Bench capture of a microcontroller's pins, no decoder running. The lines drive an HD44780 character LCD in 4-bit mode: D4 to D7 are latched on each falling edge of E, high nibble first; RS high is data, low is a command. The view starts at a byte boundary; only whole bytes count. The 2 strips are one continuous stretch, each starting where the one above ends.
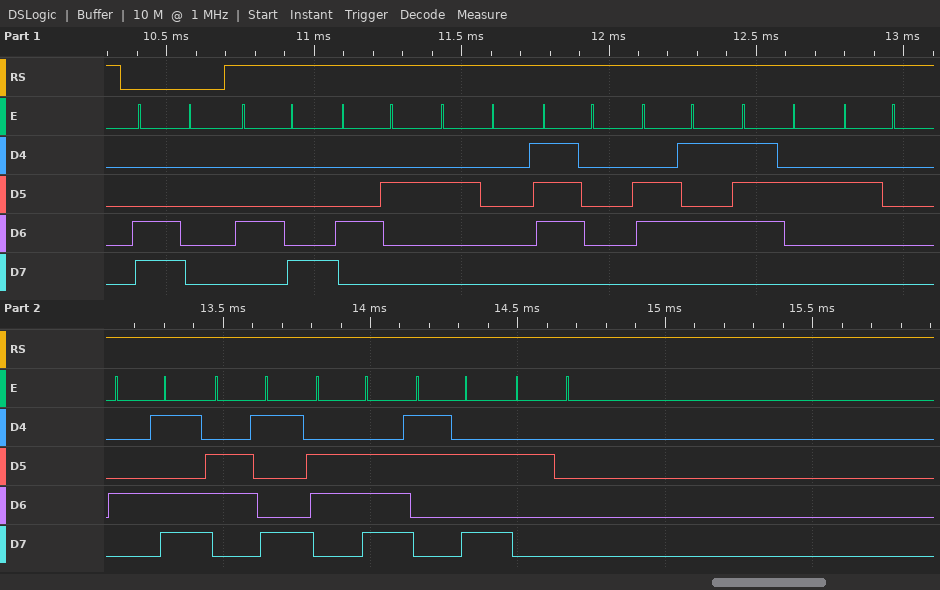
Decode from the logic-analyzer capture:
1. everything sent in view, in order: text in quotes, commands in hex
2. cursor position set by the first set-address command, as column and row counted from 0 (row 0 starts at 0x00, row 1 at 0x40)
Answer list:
0xC0 "HB per Min: "
column 0, row 1
